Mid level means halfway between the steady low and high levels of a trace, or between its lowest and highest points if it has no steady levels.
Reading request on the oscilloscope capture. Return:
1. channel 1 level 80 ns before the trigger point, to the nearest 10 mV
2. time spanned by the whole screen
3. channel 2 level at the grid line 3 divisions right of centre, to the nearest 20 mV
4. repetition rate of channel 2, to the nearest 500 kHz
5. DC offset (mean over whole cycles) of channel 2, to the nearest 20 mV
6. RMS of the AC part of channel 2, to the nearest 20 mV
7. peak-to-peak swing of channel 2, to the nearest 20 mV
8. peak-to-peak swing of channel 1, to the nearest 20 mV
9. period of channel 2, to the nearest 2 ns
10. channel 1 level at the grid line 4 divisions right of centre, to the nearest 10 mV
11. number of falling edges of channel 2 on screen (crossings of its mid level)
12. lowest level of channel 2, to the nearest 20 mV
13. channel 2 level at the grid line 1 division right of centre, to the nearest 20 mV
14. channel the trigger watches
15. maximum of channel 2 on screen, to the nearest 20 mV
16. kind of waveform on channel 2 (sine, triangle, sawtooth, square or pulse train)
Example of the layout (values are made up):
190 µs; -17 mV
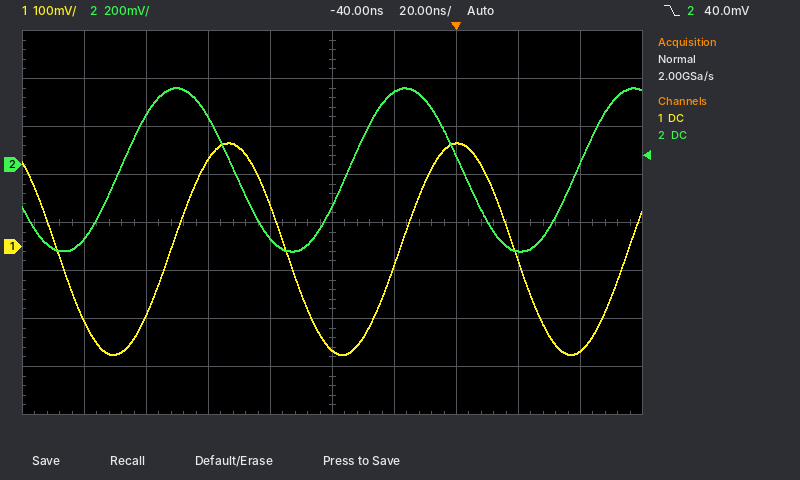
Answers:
180 mV; 200 ns; -360 mV; 13.5 MHz; -20 mV; 240 mV; 680 mV; 440 mV; 74 ns; -220 mV; 2; -360 mV; 300 mV; channel 2; 320 mV; sine
